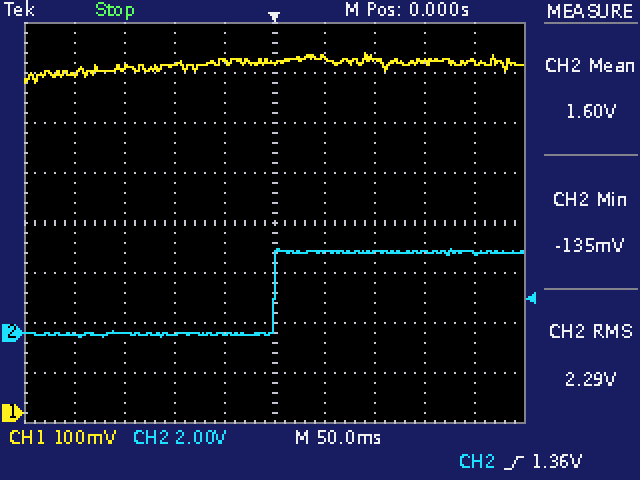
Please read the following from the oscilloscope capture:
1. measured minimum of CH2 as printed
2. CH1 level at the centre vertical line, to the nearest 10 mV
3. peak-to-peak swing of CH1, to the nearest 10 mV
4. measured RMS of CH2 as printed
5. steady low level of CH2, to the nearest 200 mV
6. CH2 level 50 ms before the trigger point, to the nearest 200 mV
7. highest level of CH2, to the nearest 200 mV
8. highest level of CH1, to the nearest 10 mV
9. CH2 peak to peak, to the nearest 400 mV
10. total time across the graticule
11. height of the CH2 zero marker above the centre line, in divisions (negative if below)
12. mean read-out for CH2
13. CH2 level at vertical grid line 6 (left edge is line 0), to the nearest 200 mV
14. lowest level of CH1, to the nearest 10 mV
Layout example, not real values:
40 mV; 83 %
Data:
-135 mV; 700 mV; 60 mV; 2.29 V; 0.0 V; 0.0 V; 3.4 V; 720 mV; 3.6 V; 500 ms; -2.2 div; 1.60 V; 3.2 V; 660 mV
